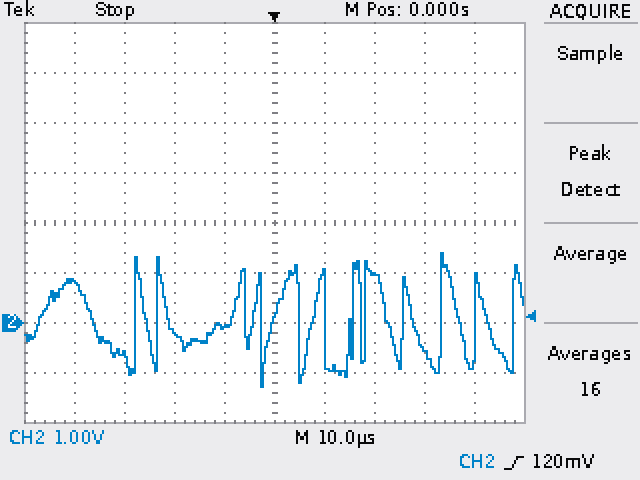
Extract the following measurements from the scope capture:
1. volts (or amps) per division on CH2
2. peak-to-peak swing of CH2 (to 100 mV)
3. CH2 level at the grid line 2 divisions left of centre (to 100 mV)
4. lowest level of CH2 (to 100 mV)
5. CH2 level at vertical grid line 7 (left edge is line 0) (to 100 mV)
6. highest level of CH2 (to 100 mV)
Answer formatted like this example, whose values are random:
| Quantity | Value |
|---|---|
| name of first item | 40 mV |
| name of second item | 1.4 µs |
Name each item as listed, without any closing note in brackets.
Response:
| Quantity | Value |
|---|---|
| volts (or amps) per division on CH2 | 1 V |
| peak-to-peak swing of CH2 | 2.7 V |
| CH2 level at the grid line 2 divisions left of centre | -200 mV |
| lowest level of CH2 | -1.3 V |
| CH2 level at vertical grid line 7 (left edge is line 0) | 1.0 V |
| highest level of CH2 | 1.4 V |
